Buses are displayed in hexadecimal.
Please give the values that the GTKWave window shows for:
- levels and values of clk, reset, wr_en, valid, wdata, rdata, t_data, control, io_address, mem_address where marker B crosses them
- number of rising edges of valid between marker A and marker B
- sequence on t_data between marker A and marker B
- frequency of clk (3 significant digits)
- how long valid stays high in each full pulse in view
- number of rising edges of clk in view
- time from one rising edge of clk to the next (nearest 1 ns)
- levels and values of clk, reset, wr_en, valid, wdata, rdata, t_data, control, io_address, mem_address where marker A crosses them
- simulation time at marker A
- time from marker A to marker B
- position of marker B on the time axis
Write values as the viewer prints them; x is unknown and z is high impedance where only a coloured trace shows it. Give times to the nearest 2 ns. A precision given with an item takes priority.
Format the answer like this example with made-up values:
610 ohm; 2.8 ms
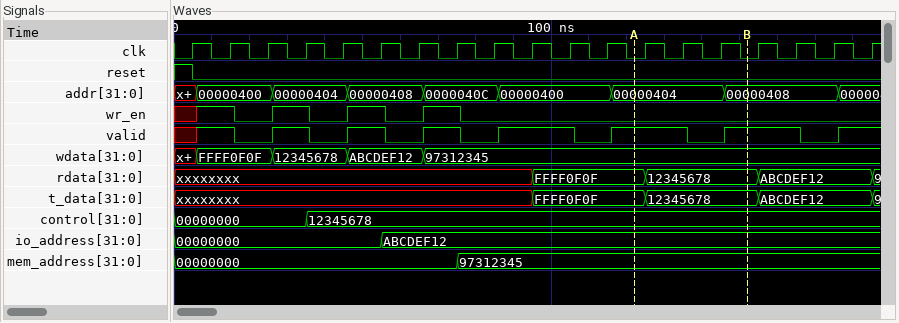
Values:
clk=0, reset=0, wr_en=0, valid=1, wdata=97312345, rdata=12345678, t_data=12345678, control=12345678, io_address=ABCDEF12, mem_address=97312345; 1; FFFF0F0F, 12345678; 100 MHz; 10 ns, 10 ns, 10 ns, 20 ns, 20 ns, 20 ns; 19; 10 ns; clk=0, reset=0, wr_en=0, valid=1, wdata=97312345, rdata=FFFF0F0F, t_data=FFFF0F0F, control=12345678, io_address=ABCDEF12, mem_address=97312345; 122 ns; 30 ns; 152 ns
